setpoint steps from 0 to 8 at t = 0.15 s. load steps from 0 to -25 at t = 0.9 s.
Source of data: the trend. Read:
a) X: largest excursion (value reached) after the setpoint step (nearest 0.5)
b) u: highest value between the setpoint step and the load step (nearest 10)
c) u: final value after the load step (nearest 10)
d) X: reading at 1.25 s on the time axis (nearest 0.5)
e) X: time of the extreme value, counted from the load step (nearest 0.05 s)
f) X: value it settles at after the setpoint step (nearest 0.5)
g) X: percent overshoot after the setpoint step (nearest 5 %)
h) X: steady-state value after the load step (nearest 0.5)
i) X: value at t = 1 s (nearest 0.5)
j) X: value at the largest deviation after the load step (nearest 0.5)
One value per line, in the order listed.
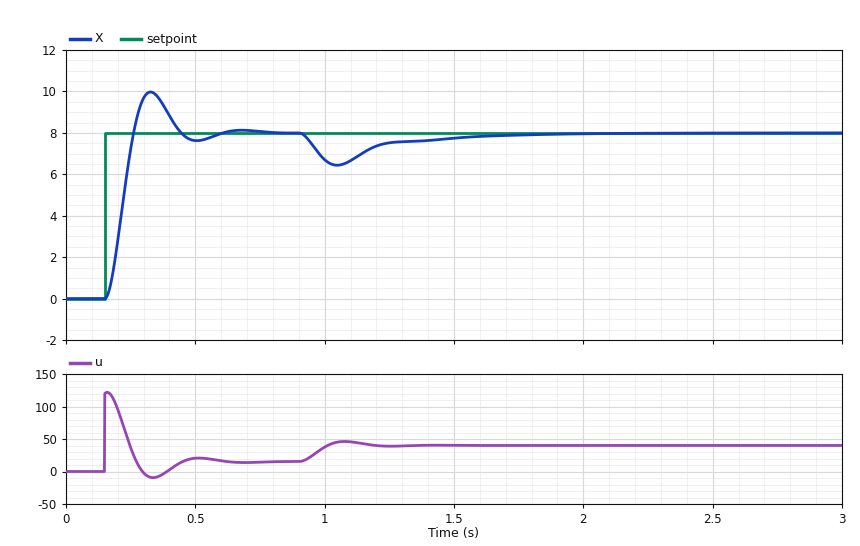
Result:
10.0
120
40
7.5
0.15 s
8.0
25 %
8.0
6.5
6.5
